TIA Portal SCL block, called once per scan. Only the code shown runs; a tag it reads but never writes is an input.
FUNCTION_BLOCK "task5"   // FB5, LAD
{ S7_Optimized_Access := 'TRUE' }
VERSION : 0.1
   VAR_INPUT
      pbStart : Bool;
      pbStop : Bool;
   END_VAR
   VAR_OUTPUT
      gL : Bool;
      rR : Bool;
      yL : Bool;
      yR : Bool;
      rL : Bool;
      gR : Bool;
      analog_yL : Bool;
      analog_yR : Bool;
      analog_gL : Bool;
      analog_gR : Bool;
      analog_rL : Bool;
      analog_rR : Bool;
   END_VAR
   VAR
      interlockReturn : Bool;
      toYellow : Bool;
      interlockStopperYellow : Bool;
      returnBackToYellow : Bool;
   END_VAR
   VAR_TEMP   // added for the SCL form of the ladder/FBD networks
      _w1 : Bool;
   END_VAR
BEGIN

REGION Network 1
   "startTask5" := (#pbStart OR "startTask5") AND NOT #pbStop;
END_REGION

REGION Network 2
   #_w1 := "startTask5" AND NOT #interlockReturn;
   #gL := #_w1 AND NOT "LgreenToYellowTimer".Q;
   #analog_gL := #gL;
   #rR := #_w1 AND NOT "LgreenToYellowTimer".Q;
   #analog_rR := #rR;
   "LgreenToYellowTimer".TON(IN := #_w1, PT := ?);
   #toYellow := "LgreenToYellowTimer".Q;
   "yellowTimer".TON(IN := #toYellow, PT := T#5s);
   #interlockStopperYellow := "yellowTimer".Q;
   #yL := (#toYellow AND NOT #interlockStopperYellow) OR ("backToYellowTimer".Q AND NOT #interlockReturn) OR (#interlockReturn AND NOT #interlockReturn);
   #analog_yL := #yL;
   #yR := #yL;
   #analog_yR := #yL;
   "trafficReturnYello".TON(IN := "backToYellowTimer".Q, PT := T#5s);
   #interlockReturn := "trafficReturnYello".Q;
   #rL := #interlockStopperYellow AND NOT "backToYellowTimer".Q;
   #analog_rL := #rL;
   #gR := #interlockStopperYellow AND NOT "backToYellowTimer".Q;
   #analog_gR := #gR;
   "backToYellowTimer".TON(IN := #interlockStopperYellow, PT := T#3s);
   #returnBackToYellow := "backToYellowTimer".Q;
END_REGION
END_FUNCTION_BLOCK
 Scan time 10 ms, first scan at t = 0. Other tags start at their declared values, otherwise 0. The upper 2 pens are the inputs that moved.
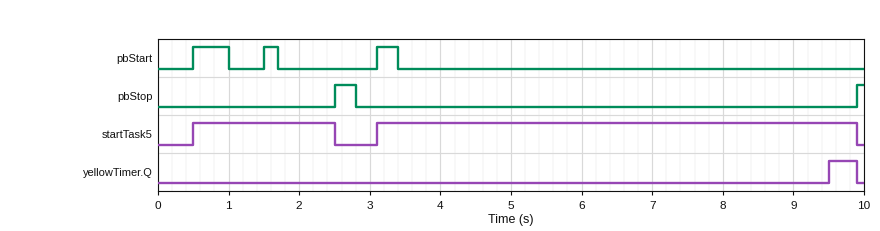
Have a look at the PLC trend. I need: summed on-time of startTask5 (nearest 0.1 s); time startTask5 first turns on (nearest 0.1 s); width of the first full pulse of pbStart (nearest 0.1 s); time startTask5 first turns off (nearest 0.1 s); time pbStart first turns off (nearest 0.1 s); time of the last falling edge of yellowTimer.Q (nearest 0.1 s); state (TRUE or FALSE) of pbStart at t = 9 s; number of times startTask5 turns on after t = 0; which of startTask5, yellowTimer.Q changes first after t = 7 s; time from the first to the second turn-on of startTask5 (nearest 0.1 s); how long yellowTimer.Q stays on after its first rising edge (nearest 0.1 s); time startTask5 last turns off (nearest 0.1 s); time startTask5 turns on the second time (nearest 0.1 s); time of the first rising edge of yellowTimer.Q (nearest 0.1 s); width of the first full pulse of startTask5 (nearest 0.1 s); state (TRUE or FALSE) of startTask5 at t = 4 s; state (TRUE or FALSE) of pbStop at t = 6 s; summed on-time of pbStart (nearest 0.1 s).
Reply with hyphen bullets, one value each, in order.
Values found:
- 8.8 s
- 0.5 s
- 0.5 s
- 2.5 s
- 1.0 s
- 9.9 s
- FALSE
- 2
- yellowTimer.Q
- 2.6 s
- 0.4 s
- 9.9 s
- 3.1 s
- 9.5 s
- 2.0 s
- TRUE
- FALSE
- 1.0 s
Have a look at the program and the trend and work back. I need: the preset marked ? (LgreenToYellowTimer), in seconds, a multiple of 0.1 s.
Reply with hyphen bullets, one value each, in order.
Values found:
- 1.4 s
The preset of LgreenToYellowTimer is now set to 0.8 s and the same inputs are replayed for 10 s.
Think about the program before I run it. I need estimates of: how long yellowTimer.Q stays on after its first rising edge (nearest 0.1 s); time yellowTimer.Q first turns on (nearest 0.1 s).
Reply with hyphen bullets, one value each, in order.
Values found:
- 1.0 s
- 8.9 s
